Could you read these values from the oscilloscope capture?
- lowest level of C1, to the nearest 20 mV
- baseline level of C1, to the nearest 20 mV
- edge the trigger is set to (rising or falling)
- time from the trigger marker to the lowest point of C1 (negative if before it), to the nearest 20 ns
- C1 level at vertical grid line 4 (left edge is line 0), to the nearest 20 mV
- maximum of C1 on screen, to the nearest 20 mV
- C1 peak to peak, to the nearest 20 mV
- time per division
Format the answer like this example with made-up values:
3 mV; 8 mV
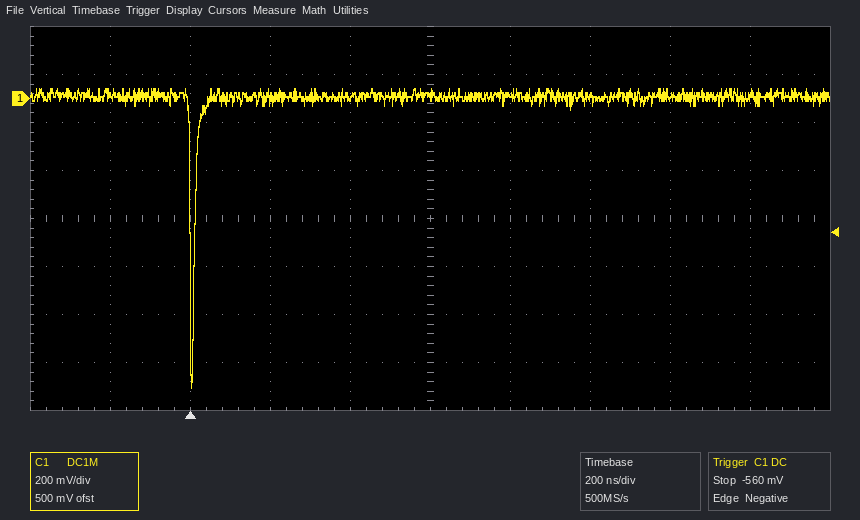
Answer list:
-1.20 V; 0 mV; falling; 0 ns; 0 mV; 40 mV; 1.24 V; 200 ns
